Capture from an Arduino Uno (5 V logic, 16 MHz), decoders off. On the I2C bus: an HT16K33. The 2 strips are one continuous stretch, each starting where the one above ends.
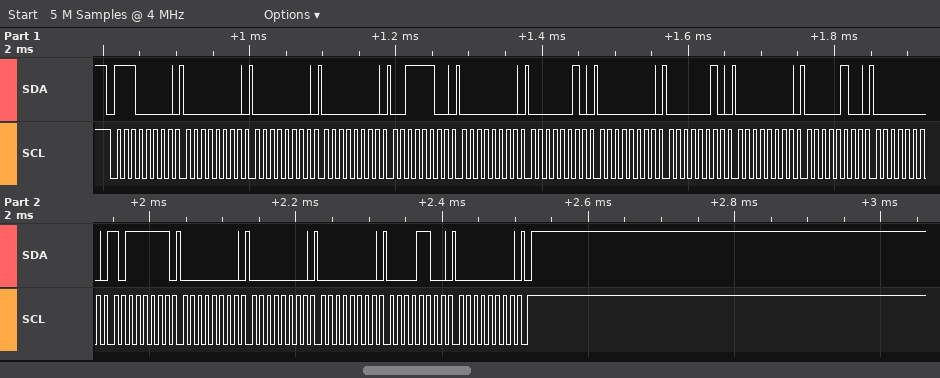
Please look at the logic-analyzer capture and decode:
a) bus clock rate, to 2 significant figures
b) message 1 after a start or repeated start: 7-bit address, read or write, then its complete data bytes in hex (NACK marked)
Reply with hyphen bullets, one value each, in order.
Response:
- 100 kHz
- 0x70 write: 00 00 00 3C 00 02 00 02 00 04 00 BF 00 00 00 0C 00
